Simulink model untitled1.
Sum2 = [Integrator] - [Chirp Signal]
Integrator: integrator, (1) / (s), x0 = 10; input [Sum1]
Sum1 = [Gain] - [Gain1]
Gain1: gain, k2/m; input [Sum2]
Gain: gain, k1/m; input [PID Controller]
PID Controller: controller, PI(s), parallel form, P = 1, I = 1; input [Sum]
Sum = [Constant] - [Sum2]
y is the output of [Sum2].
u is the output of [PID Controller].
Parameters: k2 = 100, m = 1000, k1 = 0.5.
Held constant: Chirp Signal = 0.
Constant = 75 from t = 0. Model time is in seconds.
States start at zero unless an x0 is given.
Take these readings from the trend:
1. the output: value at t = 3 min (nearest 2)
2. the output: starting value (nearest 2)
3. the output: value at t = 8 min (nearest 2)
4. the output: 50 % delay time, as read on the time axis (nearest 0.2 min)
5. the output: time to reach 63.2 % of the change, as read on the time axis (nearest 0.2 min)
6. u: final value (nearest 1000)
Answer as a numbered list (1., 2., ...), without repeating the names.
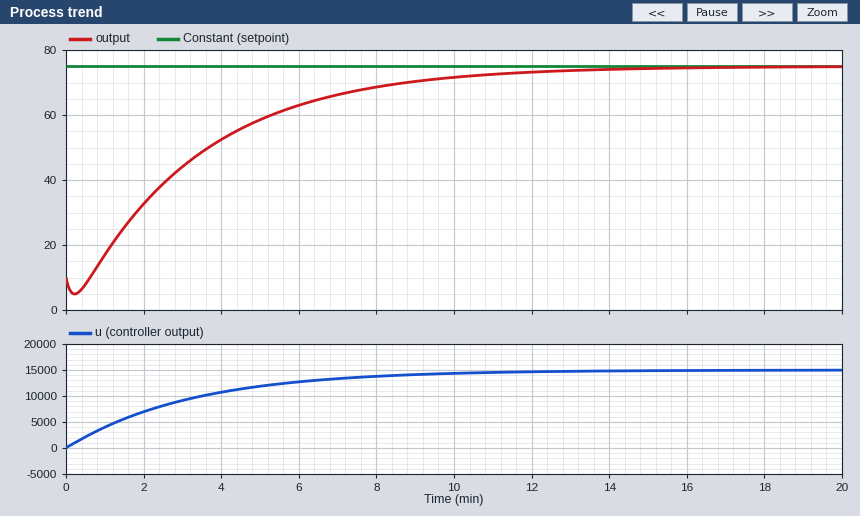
1. 44
2. 10
3. 68
4. 2.8 min
5. 3.8 min
6. 15000
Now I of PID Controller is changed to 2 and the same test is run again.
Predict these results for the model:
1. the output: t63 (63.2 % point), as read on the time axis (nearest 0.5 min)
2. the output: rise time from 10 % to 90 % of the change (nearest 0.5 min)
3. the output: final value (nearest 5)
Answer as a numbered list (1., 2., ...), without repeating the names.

1. 2.0 min
2. 3.5 min
3. 75
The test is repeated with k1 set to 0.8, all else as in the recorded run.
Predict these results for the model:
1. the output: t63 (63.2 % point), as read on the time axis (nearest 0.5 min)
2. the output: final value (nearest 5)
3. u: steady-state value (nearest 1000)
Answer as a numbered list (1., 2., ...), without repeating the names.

1. 2.5 min
2. 75
3. 9000
